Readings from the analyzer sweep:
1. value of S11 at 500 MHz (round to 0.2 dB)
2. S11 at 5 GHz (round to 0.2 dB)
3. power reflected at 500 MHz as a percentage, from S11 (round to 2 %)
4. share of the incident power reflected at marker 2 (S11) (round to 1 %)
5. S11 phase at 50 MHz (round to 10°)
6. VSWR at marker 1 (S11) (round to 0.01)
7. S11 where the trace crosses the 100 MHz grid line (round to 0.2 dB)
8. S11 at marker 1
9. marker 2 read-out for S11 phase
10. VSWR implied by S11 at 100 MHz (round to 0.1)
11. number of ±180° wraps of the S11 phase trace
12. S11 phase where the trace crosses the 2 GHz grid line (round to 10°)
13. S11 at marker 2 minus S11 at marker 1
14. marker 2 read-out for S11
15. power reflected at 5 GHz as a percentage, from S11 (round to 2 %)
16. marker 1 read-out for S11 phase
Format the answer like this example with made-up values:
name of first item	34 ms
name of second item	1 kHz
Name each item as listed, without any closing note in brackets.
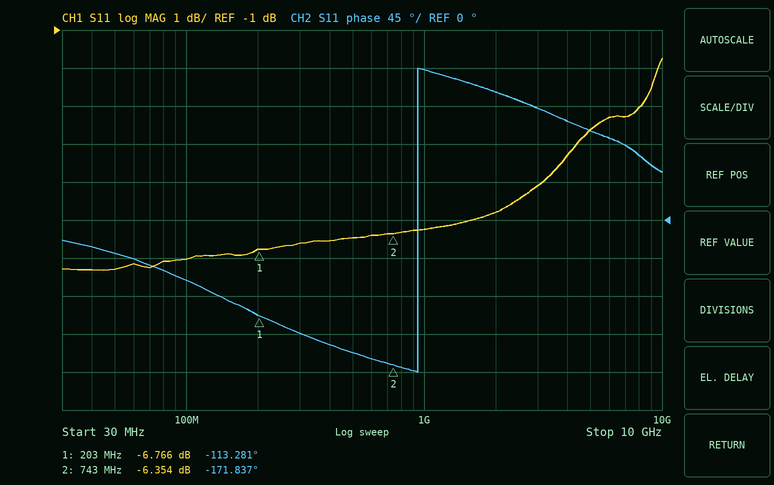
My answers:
value of S11 at 500 MHz	-6.4 dB
S11 at 5 GHz	-3.6 dB
power reflected at 500 MHz as a percentage, from S11	22 %
share of the incident power reflected at marker 2 (S11)	23 %
S11 phase at 50 MHz	-40°
VSWR at marker 1 (S11)	2.70
S11 where the trace crosses the 100 MHz grid line	-7.0 dB
S11 at marker 1	-6.766 dB
marker 2 read-out for S11 phase	-171.837°
VSWR implied by S11 at 100 MHz	2.6
number of ±180° wraps of the S11 phase trace	1
S11 phase where the trace crosses the 2 GHz grid line	150°
S11 at marker 2 minus S11 at marker 1	0.412 dB
marker 2 read-out for S11	-6.354 dB
power reflected at 5 GHz as a percentage, from S11	44 %
marker 1 read-out for S11 phase	-113.281°
